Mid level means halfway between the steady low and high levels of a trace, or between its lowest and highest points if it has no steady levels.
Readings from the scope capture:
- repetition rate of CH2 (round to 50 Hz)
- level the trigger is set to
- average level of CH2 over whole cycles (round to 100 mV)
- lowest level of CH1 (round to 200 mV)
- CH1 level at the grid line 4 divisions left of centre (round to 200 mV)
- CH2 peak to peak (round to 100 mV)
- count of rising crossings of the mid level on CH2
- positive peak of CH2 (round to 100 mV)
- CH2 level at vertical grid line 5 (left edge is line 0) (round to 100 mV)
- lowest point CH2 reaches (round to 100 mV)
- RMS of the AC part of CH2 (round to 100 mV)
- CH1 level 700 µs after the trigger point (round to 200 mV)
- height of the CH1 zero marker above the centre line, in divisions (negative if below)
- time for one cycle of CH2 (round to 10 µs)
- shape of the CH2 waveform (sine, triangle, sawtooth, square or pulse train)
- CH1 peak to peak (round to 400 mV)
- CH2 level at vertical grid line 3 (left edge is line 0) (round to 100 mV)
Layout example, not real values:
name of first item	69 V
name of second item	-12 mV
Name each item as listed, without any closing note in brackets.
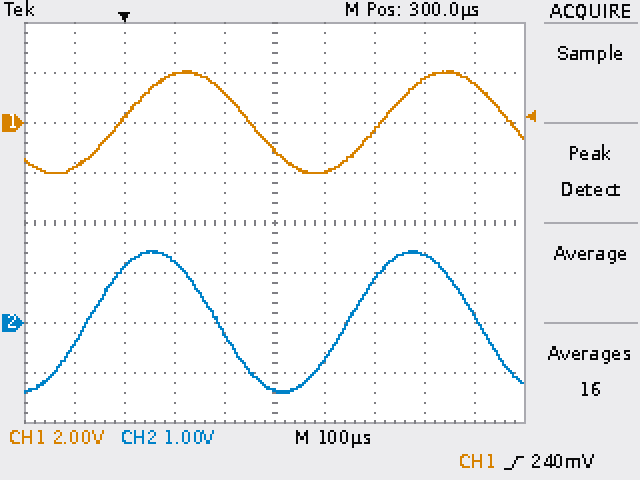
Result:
repetition rate of CH2	1.90 kHz
level the trigger is set to	240 mV
average level of CH2 over whole cycles	0.0 V
lowest level of CH1	-2.0 V
CH1 level at the grid line 4 divisions left of centre	-1.8 V
CH2 peak to peak	2.8 V
count of rising crossings of the mid level on CH2	2
positive peak of CH2	1.4 V
CH2 level at vertical grid line 5 (left edge is line 0)	-1.4 V
lowest point CH2 reaches	-1.4 V
RMS of the AC part of CH2	1.0 V
CH1 level 700 µs after the trigger point	1.6 V
height of the CH1 zero marker above the centre line, in divisions	+2.0 div
time for one cycle of CH2	520 µs
shape of the CH2 waveform	sine
CH1 peak to peak	4.0 V
CH2 level at vertical grid line 3 (left edge is line 0)	1.2 V
